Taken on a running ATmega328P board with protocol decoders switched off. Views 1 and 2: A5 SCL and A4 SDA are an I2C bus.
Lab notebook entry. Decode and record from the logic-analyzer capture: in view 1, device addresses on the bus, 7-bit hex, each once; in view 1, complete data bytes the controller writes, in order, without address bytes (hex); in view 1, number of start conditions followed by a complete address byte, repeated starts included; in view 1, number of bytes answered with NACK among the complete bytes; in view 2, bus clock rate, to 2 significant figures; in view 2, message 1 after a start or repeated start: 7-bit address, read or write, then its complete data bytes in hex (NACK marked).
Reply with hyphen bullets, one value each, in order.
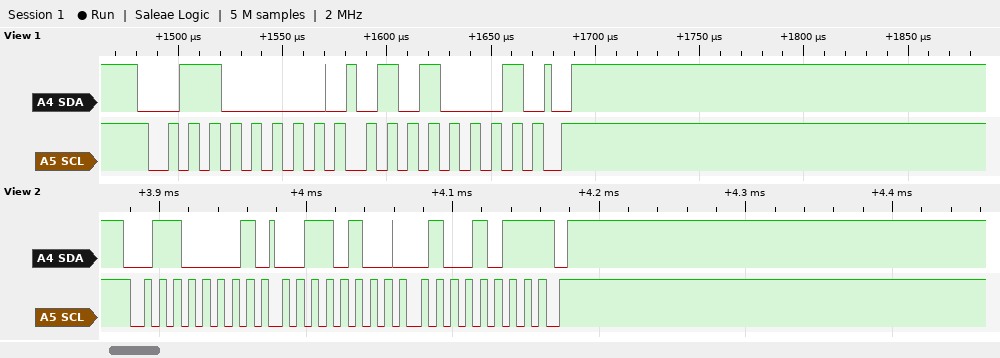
- 0x30
- 51
- 1
- 0
- 100 kHz
- 0x30 read: 34 4B NACK
